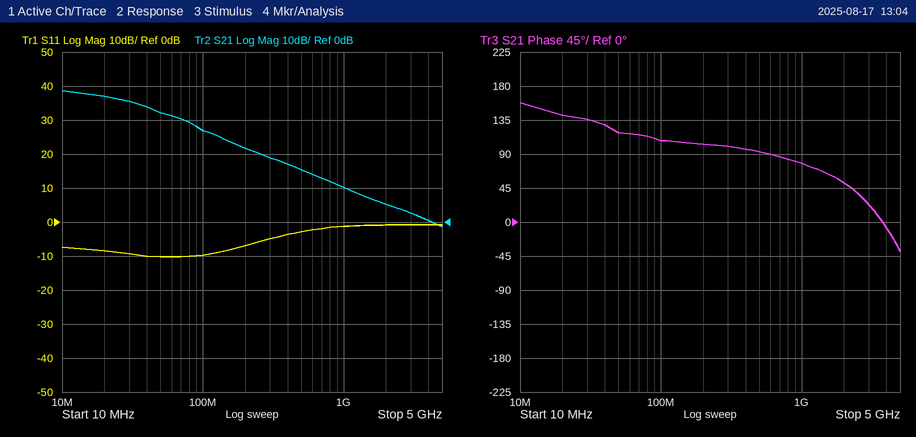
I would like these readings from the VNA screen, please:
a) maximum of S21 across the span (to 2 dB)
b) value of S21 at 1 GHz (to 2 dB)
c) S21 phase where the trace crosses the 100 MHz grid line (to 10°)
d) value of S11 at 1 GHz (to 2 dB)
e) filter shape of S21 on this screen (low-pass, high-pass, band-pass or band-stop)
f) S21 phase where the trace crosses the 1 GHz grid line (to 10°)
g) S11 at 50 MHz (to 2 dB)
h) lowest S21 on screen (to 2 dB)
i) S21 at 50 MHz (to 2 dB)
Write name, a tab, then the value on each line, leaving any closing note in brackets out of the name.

maximum of S21 across the span	38 dB
value of S21 at 1 GHz	10 dB
S21 phase where the trace crosses the 100 MHz grid line	110°
value of S11 at 1 GHz	-2 dB
filter shape of S21 on this screen	low-pass
S21 phase where the trace crosses the 1 GHz grid line	80°
S11 at 50 MHz	-10 dB
lowest S21 on screen	-2 dB
S21 at 50 MHz	32 dB
